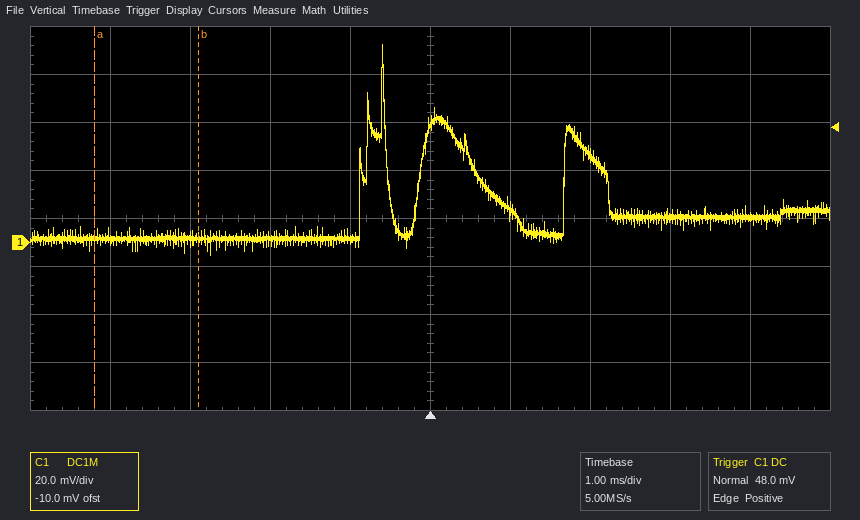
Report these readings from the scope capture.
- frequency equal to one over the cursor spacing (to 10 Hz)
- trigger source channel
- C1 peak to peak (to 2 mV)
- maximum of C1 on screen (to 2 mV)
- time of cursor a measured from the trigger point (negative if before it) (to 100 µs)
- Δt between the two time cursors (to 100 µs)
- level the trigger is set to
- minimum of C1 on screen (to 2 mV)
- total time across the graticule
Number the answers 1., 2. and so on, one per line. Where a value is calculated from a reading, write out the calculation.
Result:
1. 1 / 1.3 ms ≈ 770 Hz
2. C1
3. 82 mV − (-6 mV) = 88 mV
4. 82 mV
5. -4.2 ms
6. 1.3 ms
7. 48.0 mV
8. -6 mV
9. 10 ms
